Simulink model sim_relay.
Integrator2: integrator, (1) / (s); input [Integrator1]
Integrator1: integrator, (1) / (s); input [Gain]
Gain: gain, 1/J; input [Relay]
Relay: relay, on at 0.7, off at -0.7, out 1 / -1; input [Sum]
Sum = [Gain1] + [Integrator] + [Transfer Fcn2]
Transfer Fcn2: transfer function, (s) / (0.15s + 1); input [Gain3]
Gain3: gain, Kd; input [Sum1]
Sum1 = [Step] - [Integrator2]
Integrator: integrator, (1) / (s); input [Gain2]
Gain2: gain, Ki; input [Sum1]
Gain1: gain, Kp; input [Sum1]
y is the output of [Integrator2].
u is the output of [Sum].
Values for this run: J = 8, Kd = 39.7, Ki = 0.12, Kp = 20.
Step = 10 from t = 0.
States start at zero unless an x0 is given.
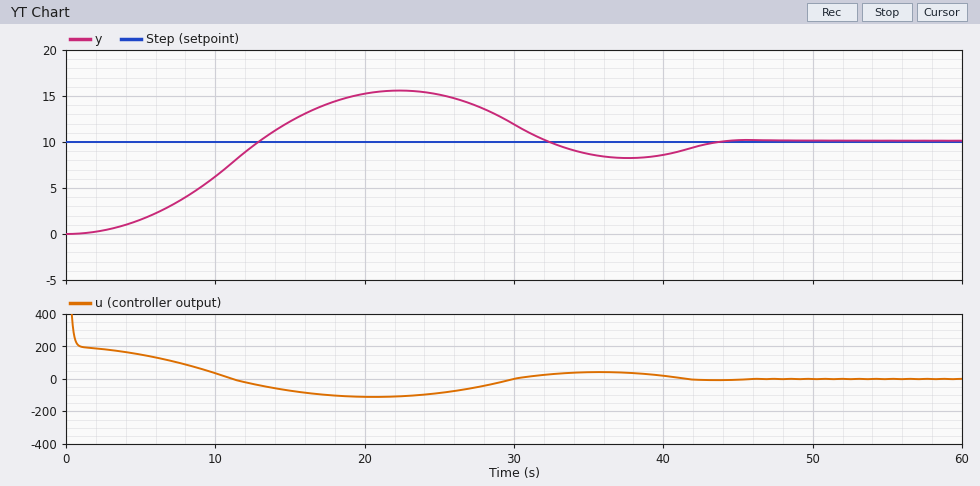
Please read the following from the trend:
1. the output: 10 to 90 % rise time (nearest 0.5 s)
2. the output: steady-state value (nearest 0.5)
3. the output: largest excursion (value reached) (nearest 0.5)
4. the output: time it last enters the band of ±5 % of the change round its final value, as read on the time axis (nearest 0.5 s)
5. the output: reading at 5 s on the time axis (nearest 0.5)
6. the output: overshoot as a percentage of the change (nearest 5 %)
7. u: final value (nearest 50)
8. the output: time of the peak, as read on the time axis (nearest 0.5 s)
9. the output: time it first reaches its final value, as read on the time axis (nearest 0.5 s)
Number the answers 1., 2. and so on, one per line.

1. 8.0 s
2. 10.0
3. 15.5
4. 42.5 s
5. 1.5
6. 55 %
7. 0
8. 22.5 s
9. 13.0 s
